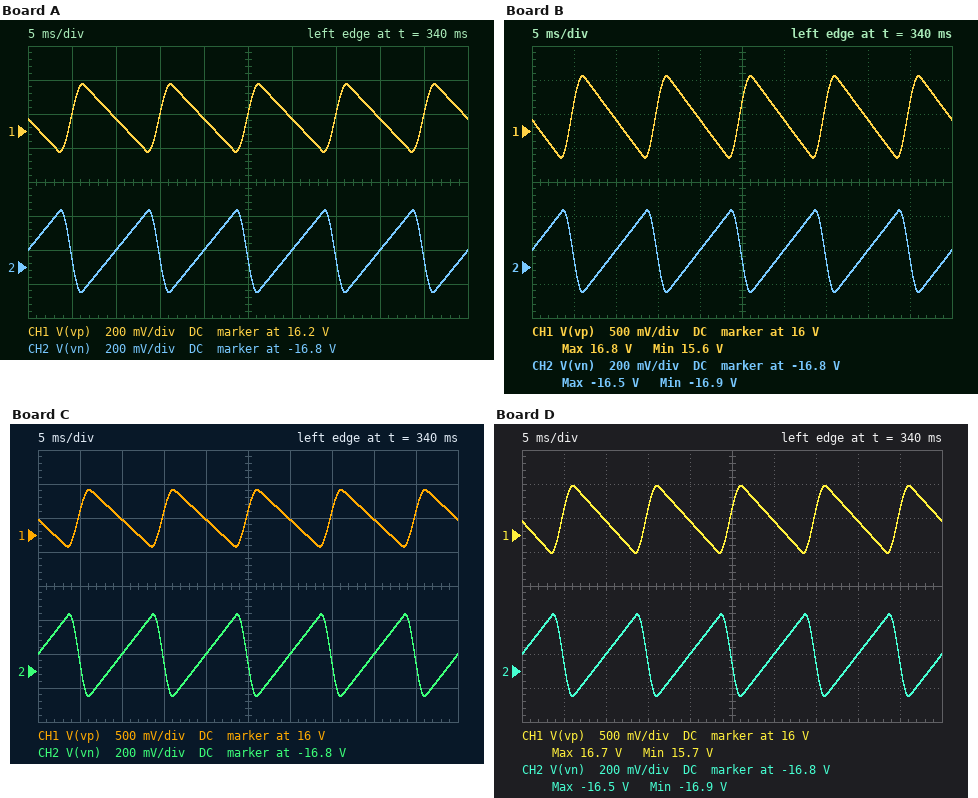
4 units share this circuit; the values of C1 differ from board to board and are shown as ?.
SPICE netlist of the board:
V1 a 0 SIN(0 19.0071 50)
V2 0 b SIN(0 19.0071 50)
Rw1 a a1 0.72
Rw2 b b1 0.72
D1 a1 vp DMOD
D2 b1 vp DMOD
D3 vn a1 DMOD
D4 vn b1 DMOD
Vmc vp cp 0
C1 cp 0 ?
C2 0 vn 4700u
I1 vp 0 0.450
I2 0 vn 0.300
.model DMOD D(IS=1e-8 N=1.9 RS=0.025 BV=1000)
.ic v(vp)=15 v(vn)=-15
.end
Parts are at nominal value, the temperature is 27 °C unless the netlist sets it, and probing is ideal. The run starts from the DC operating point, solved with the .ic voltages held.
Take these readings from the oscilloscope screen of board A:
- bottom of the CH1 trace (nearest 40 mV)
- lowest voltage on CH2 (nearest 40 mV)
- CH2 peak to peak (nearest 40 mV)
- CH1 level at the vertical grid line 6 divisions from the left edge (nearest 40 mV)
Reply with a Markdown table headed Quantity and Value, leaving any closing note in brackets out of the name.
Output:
| Quantity | Value |
|---|---|
| bottom of the CH1 trace | 16.08 V |
| lowest voltage on CH2 | -16.96 V |
| CH2 peak to peak | 480 mV |
| CH1 level at the vertical grid line 6 divisions from the left edge | 16.28 V |
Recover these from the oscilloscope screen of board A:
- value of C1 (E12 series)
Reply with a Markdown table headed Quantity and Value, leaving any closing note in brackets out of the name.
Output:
| Quantity | Value |
|---|---|
| value of C1 | 8.2 mF |
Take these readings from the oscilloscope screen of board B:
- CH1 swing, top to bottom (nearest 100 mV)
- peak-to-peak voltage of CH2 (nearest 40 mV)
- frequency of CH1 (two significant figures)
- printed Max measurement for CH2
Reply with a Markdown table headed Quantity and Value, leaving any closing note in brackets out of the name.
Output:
| Quantity | Value |
|---|---|
| CH1 swing, top to bottom | 1.2 V |
| peak-to-peak voltage of CH2 | 480 mV |
| frequency of CH1 | 100 Hz |
| printed Max measurement for CH2 | -16.5 V |
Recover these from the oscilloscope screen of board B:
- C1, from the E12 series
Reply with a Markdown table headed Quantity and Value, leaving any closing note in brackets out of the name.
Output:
| Quantity | Value |
|---|---|
| C1, from the E12 series | 2.7 mF |
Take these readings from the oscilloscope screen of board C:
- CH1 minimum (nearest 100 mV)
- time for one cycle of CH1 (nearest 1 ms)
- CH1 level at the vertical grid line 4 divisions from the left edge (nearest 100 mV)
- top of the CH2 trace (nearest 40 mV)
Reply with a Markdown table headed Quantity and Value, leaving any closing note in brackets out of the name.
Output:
| Quantity | Value |
|---|---|
| CH1 minimum | 15.8 V |
| time for one cycle of CH1 | 10 ms |
| CH1 level at the vertical grid line 4 divisions from the left edge | 16.2 V |
| top of the CH2 trace | -16.48 V |
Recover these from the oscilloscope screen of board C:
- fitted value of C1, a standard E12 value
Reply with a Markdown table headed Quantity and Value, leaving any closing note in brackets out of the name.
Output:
| Quantity | Value |
|---|---|
| fitted value of C1, a standard E12 value | 3.9 mF |
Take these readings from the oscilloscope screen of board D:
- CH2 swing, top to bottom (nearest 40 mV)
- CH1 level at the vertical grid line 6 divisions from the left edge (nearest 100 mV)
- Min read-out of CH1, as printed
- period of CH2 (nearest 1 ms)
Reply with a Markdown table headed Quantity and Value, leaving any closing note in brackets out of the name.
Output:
| Quantity | Value |
|---|---|
| CH2 swing, top to bottom | 480 mV |
| CH1 level at the vertical grid line 6 divisions from the left edge | 16.2 V |
| Min read-out of CH1, as printed | 15.7 V |
| period of CH2 | 10 ms |
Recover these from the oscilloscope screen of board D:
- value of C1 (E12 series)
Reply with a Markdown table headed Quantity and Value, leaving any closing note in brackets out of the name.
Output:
| Quantity | Value |
|---|---|
| value of C1 | 3.3 mF |
